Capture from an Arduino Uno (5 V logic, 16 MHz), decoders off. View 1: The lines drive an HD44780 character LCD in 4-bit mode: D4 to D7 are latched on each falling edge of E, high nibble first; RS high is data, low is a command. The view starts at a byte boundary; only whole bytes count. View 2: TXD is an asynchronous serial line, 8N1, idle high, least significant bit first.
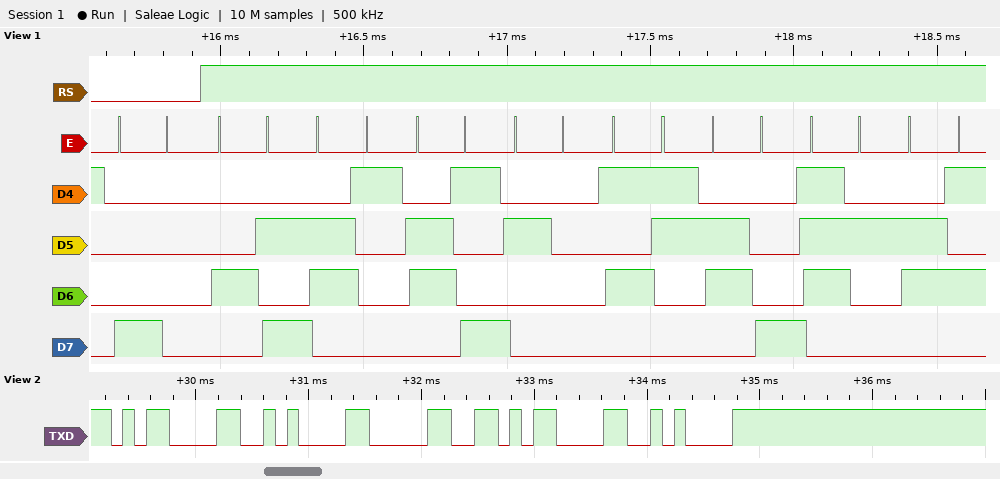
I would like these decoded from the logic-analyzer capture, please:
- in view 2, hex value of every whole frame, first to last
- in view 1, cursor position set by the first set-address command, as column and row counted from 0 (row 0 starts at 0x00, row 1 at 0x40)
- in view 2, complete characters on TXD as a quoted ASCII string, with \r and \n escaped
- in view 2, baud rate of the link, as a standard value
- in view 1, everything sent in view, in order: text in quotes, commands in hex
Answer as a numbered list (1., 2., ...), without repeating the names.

1. 0D 0A 30 0D 0A
2. column 0, row 0
3. "\r\n0\r\n"
4. 9600 baud
5. 0x80 "Jai Shre"
